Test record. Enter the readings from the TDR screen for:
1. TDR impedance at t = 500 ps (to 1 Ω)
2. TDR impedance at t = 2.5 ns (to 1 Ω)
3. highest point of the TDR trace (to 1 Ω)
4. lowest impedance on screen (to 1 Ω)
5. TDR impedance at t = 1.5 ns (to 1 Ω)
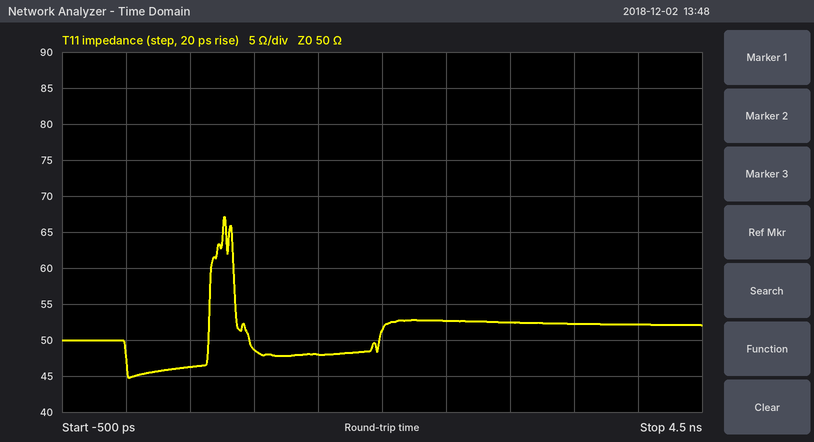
46 Ω
53 Ω
67 Ω
45 Ω
48 Ω
